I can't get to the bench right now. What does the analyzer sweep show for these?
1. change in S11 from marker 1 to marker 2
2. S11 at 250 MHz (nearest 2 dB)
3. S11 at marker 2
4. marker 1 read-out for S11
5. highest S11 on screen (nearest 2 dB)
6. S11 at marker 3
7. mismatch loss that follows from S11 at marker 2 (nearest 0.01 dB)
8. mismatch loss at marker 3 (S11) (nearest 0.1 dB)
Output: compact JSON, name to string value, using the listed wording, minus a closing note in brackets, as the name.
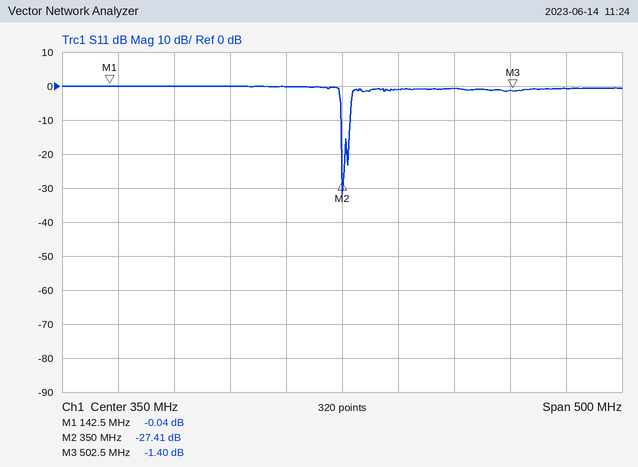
{"change in S11 from marker 1 to marker 2": "-27.37 dB", "S11 at 250 MHz": "0 dB", "S11 at marker 2": "-27.41 dB", "marker 1 read-out for S11": "-0.04 dB", "highest S11 on screen": "0 dB", "S11 at marker 3": "-1.40 dB", "mismatch loss that follows from S11 at marker 2": "0.01 dB", "mismatch loss at marker 3 (S11)": "5.6 dB"}
